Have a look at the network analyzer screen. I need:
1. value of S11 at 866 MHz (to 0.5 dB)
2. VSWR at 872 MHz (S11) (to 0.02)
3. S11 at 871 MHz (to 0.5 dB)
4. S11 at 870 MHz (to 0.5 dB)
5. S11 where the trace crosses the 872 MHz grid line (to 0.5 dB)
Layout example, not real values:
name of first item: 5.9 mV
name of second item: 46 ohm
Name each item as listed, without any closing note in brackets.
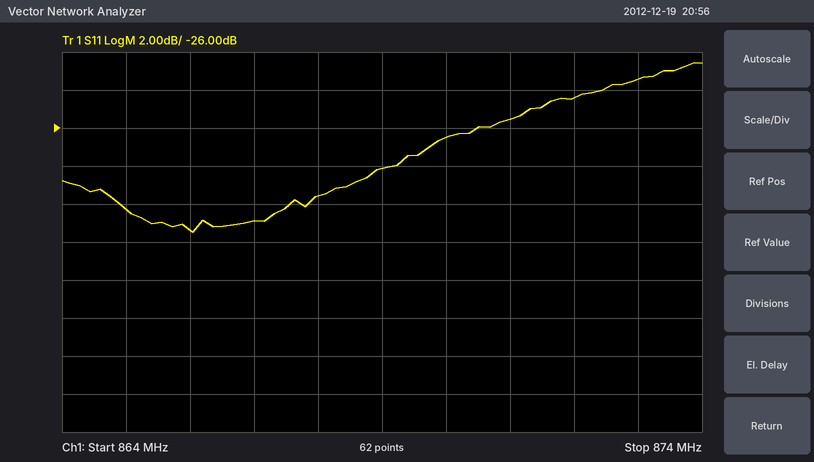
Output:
value of S11 at 866 MHz: -31.5 dB
VSWR at 872 MHz (S11): 1.12
S11 at 871 MHz: -25.5 dB
S11 at 870 MHz: -26.5 dB
S11 where the trace crosses the 872 MHz grid line: -24.5 dB
